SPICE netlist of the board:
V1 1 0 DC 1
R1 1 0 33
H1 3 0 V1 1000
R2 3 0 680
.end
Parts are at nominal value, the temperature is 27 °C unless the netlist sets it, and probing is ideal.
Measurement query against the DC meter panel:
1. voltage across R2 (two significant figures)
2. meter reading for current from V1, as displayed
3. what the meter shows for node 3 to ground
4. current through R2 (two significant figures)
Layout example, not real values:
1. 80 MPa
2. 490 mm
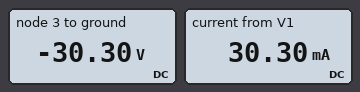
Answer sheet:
1. 30 V
2. 30.30 mA
3. -30.30 V
4. 45 mA
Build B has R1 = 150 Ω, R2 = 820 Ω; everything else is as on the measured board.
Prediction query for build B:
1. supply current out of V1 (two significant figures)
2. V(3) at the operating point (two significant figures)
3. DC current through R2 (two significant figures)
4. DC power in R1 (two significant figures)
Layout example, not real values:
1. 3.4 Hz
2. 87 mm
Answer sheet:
1. 6.7 mA
2. -6.7 V
3. 8.1 mA
4. 6.7 mW
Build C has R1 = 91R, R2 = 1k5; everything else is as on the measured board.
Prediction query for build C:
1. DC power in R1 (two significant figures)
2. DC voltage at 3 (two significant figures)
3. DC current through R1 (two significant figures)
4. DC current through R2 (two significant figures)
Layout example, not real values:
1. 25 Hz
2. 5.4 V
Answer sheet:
1. 11 mW
2. -11 V
3. 11 mA
4. 7.3 mA
